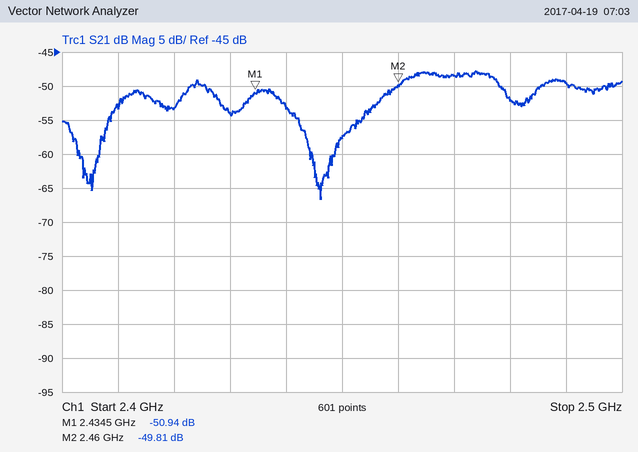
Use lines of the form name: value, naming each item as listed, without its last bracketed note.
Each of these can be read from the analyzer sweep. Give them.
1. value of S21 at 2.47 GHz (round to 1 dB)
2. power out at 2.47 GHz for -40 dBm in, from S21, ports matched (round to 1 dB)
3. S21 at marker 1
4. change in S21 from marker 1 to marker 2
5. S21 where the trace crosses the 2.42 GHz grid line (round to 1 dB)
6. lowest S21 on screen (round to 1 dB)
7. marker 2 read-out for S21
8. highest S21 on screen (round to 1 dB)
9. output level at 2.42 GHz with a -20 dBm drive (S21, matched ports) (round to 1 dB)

value of S21 at 2.47 GHz: -48 dB
power out at 2.47 GHz for -40 dBm in, from S21, ports matched: -88 dBm
S21 at marker 1: -50.94 dB
change in S21 from marker 1 to marker 2: 1.13 dB
S21 where the trace crosses the 2.42 GHz grid line: -53 dB
lowest S21 on screen: -67 dB
marker 2 read-out for S21: -49.81 dB
highest S21 on screen: -48 dB
output level at 2.42 GHz with a -20 dBm drive (S21, matched ports): -73 dBm
